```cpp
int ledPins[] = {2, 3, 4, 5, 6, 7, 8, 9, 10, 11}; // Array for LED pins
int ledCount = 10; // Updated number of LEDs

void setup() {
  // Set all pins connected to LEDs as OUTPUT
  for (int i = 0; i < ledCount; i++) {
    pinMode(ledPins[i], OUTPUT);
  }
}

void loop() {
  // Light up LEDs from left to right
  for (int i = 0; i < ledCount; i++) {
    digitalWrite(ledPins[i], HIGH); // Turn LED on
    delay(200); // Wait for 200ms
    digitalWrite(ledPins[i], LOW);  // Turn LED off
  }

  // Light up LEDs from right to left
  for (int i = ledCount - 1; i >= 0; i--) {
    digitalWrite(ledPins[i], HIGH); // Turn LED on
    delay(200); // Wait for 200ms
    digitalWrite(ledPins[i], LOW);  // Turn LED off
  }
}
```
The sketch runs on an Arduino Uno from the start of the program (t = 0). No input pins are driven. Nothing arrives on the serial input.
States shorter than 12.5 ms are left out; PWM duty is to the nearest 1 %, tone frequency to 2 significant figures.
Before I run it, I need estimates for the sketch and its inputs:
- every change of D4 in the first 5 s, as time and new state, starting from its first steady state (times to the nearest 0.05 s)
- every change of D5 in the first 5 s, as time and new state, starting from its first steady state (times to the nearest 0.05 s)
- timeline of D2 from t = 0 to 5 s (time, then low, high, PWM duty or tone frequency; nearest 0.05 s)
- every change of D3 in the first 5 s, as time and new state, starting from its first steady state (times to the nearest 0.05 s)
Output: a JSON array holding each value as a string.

["0 s low; 0.4 s high; 0.6 s low; 3.4 s high; 3.6 s low; 4.4 s high; 4.6 s low", "0 s low; 0.6 s high; 0.8 s low; 3.2 s high; 3.4 s low; 4.6 s high; 4.8 s low", "0 s high; 0.2 s low; 3.8 s high; 4.2 s low", "0 s low; 0.2 s high; 0.4 s low; 3.6 s high; 3.8 s low; 4.2 s high; 4.4 s low"]
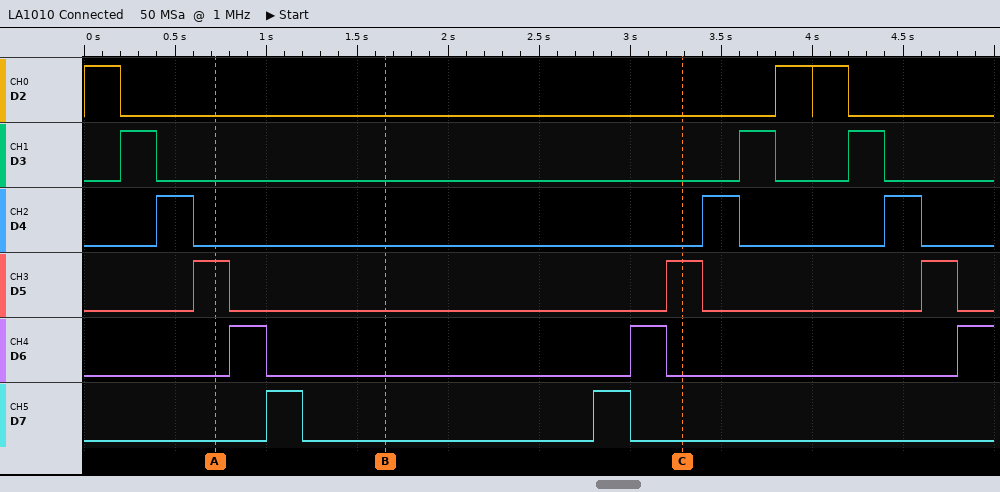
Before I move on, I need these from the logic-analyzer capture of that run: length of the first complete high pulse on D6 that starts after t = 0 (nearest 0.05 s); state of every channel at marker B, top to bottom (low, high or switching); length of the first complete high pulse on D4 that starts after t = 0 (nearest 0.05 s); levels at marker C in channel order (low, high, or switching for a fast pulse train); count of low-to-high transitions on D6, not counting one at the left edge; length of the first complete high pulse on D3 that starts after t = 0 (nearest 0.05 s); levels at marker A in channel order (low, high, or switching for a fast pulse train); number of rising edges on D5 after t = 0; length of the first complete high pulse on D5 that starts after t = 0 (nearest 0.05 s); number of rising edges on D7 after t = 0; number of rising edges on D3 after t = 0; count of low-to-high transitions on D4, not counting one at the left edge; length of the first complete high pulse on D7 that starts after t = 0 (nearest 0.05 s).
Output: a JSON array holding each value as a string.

["0.20 s", "D2 low, D3 low, D4 low, D5 low, D6 low, D7 low", "0.20 s", "D2 low, D3 low, D4 low, D5 high, D6 low, D7 low", "3", "0.20 s", "D2 low, D3 low, D4 low, D5 high, D6 low, D7 low", "3", "0.20 s", "2", "3", "3", "0.20 s"]
